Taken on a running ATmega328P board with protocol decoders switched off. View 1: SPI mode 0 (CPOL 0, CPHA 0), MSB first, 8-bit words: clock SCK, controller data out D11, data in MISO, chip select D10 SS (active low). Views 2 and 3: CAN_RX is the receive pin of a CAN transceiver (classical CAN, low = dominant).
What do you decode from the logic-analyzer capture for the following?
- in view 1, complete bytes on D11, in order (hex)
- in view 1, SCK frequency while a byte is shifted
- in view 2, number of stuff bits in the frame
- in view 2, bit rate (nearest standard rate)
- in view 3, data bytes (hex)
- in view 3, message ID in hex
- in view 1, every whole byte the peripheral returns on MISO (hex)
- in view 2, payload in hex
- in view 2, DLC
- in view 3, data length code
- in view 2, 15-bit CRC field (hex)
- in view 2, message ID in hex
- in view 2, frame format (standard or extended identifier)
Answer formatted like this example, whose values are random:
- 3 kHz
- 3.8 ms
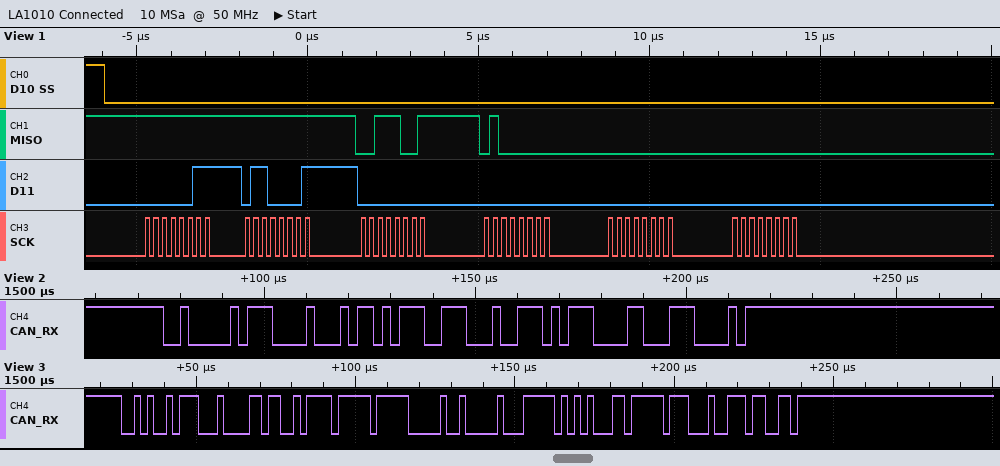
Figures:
- 03 61 00 00 00 00
- 4 MHz
- 1
- 500 kbit/s
- 6C BD FF 81 00 FD 46 FF
- 0x297
- FF FF 39 40 00 00
- 5A E7 13 AE
- 4
- 8
- 0x0C70
- 0x207
- standard
